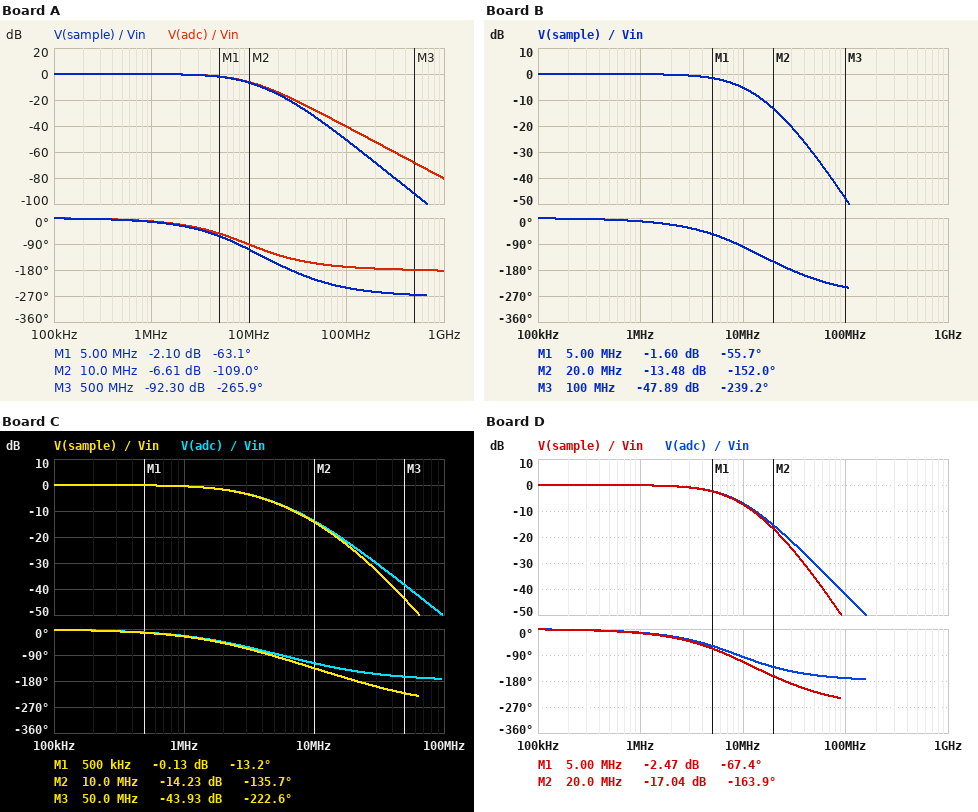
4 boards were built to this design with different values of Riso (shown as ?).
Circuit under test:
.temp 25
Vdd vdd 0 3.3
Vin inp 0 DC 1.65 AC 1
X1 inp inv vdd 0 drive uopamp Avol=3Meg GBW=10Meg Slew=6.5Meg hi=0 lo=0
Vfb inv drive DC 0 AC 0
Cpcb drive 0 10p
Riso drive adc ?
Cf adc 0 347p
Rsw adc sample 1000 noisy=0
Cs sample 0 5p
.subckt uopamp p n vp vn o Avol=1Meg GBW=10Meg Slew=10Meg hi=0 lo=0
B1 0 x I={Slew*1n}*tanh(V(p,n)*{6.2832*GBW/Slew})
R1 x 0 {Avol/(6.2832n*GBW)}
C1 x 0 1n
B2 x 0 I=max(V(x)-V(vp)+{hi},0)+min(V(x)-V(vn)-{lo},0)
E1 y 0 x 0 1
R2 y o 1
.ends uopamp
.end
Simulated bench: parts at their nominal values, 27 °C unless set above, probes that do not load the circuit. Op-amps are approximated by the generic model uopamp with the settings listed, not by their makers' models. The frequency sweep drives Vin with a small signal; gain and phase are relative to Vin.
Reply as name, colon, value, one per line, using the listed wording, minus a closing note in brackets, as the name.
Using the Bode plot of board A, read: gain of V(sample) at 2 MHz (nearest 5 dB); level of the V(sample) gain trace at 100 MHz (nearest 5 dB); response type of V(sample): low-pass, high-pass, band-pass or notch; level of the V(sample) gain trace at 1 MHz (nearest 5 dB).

gain of V(sample) at 2 MHz: 0 dB
level of the V(sample) gain trace at 100 MHz: -50 dB
response type of V(sample): low-pass, high-pass, band-pass or notch: low-pass
level of the V(sample) gain trace at 1 MHz: 0 dB
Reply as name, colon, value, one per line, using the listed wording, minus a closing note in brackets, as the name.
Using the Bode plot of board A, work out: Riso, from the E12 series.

Riso, from the E12 series: 47 Ω
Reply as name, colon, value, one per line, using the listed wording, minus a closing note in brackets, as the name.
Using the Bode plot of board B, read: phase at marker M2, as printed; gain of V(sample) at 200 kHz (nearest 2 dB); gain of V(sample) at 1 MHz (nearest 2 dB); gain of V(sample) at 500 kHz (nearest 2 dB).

phase at marker M2, as printed: -152.0 deg
gain of V(sample) at 200 kHz: 0 dB
gain of V(sample) at 1 MHz: 0 dB
gain of V(sample) at 500 kHz: 0 dB
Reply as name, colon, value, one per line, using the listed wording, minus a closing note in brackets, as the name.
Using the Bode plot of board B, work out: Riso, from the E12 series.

Riso, from the E12 series: 33 Ω
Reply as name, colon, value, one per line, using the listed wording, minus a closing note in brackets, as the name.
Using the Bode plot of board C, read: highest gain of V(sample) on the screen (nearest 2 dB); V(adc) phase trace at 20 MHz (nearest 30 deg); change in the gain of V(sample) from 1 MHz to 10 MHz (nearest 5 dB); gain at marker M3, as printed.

highest gain of V(sample) on the screen: 0 dB
V(adc) phase trace at 20 MHz: -150 deg
change in the gain of V(sample) from 1 MHz to 10 MHz: -15 dB
gain at marker M3, as printed: -43.93 dB
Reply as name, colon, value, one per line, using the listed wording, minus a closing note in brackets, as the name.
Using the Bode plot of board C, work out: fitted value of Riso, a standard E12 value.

fitted value of Riso, a standard E12 value: 150 Ω
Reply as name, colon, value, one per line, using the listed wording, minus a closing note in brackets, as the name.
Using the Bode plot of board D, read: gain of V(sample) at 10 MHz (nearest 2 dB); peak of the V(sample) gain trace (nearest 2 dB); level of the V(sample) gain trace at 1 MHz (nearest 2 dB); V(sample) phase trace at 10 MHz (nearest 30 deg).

gain of V(sample) at 10 MHz: -8 dB
peak of the V(sample) gain trace: 0 dB
level of the V(sample) gain trace at 1 MHz: 0 dB
V(sample) phase trace at 10 MHz: -120 deg
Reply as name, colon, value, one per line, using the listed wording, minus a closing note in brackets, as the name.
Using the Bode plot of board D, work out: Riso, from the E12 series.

Riso, from the E12 series: 56 Ω
